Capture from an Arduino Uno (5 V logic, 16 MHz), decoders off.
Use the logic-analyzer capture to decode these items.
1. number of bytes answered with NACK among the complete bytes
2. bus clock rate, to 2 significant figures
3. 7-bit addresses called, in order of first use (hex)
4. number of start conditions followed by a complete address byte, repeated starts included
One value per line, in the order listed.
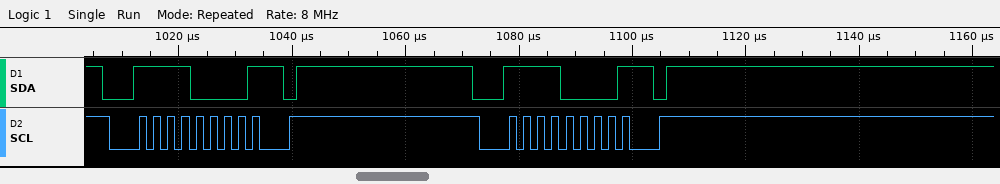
2
400 kHz
0x78
2
